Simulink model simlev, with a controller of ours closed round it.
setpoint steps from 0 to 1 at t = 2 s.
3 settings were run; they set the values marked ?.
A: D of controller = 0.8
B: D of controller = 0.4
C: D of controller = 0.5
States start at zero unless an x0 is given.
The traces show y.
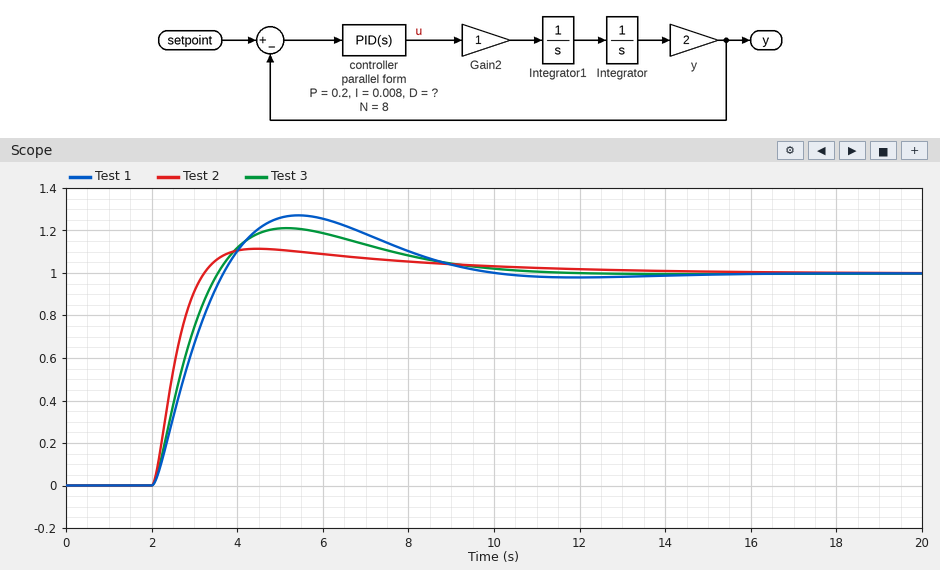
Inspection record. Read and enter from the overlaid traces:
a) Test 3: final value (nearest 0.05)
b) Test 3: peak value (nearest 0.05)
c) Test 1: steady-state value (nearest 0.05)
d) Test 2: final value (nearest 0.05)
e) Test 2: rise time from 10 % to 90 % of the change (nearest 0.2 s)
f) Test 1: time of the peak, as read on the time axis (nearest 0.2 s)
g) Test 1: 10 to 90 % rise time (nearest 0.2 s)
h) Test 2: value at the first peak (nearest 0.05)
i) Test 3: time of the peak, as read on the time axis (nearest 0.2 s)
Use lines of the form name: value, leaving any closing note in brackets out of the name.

Test 3: final value: 1.00
Test 3: peak value: 1.20
Test 1: steady-state value: 1.00
Test 2: final value: 1.00
Test 2: rise time from 10 % to 90 % of the change: 0.8 s
Test 1: time of the peak, as read on the time axis: 5.4 s
Test 1: 10 to 90 % rise time: 1.2 s
Test 2: value at the first peak: 1.10
Test 3: time of the peak, as read on the time axis: 5.2 s
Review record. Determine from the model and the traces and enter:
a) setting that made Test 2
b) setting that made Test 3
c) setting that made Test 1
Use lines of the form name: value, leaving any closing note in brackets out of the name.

setting that made Test 2: A
setting that made Test 3: C
setting that made Test 1: B
